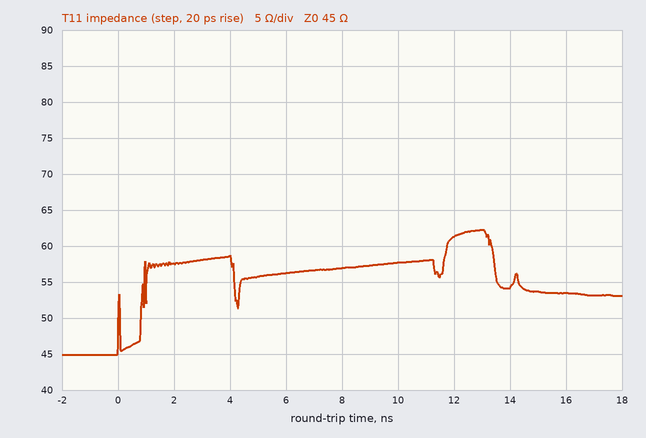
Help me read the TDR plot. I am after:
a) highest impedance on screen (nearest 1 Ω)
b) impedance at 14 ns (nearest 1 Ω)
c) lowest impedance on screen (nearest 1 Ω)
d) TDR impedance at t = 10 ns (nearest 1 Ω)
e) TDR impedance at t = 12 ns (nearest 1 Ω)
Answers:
62 Ω
54 Ω
45 Ω
58 Ω
61 Ω
